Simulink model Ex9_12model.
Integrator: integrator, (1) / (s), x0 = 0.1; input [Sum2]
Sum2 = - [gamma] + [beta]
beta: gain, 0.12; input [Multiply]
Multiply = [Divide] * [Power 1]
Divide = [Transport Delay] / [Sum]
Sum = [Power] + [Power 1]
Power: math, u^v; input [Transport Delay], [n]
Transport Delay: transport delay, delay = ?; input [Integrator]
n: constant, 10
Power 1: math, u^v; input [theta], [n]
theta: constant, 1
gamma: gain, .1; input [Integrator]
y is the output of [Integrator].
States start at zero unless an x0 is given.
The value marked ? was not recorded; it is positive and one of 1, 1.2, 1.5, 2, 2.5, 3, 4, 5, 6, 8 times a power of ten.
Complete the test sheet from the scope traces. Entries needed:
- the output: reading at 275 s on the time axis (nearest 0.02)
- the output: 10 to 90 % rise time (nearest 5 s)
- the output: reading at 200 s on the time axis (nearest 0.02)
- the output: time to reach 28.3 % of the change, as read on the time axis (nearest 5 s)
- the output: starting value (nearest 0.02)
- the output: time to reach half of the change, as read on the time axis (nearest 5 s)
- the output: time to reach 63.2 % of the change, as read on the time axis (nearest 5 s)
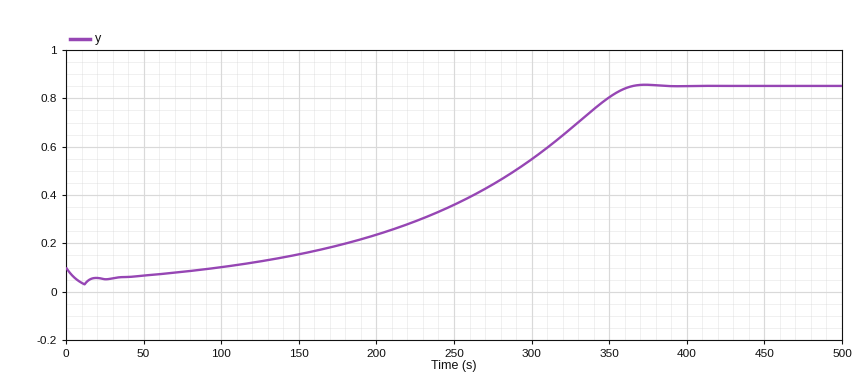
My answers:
0.44
180 s
0.24
235 s
0.10
285 s
305 s
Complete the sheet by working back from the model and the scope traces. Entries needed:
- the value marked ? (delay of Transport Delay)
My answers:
12
